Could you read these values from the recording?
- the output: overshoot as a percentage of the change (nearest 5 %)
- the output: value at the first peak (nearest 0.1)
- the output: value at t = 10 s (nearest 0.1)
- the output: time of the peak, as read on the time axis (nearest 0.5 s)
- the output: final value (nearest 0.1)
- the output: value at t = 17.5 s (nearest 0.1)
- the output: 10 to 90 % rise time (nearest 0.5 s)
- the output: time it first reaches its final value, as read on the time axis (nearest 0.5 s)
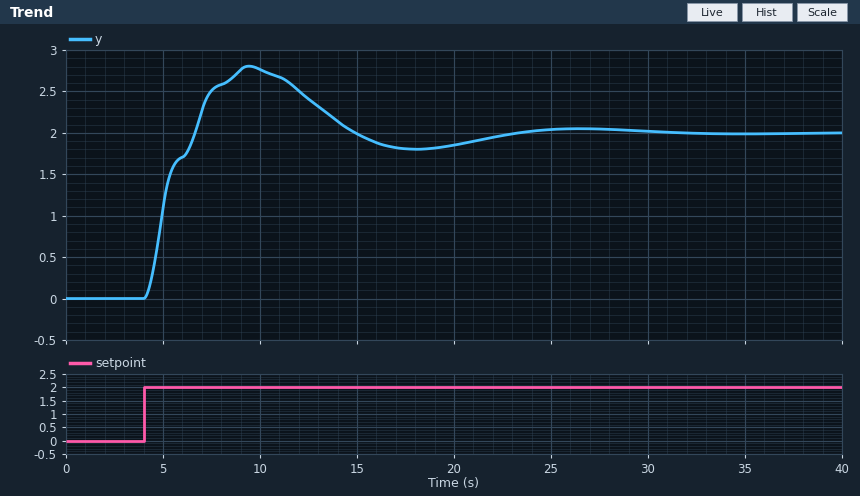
40 %
2.8
2.8
9.5 s
2.0
1.8
2.0 s
6.5 s
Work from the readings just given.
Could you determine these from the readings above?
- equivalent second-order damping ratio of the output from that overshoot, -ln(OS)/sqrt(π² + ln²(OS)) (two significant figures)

0.28
